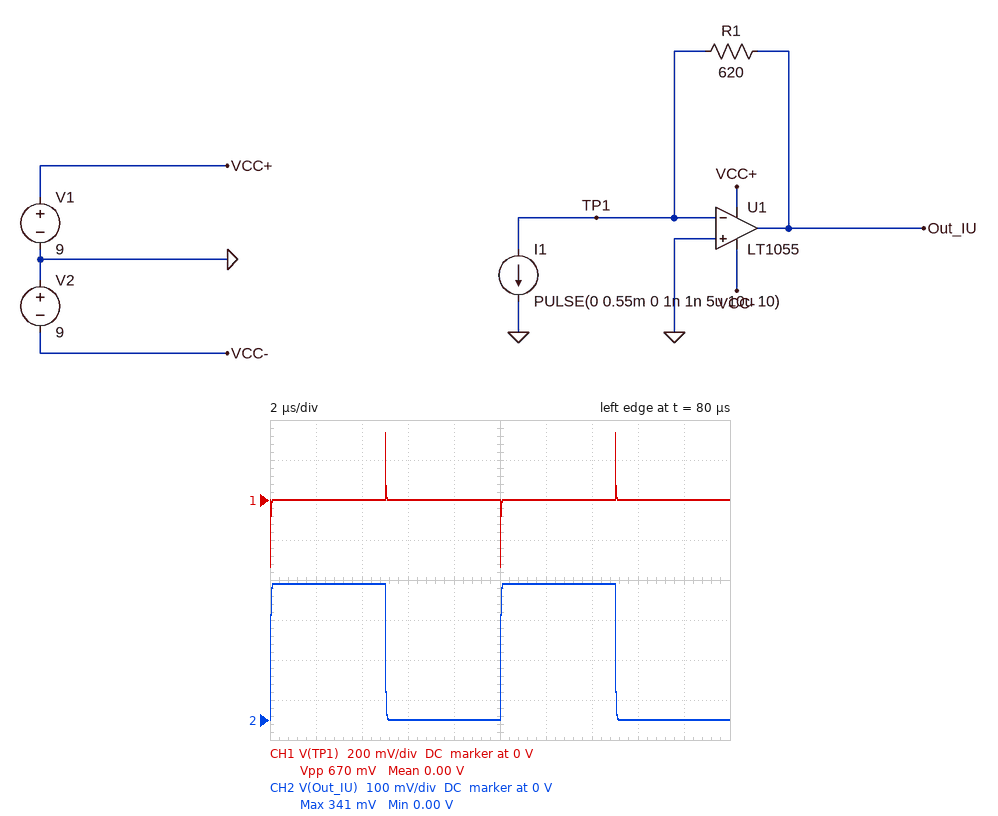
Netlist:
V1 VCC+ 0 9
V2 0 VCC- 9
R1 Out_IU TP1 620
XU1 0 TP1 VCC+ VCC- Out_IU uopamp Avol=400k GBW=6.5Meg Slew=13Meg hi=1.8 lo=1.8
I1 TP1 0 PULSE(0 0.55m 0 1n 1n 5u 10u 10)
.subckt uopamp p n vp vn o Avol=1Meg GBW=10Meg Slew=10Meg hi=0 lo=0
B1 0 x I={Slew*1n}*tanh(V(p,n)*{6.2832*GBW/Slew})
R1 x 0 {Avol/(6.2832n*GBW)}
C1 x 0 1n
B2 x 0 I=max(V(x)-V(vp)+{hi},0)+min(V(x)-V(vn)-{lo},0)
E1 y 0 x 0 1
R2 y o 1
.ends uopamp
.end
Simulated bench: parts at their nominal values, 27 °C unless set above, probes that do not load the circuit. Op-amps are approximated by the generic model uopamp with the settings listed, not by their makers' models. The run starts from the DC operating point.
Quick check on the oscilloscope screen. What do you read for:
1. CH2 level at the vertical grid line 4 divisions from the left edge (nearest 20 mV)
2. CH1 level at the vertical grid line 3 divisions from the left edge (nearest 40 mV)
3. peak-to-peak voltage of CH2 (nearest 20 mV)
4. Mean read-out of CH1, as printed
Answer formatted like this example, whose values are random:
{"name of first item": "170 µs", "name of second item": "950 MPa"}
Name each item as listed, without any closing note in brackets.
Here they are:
{"CH2 level at the vertical grid line 4 divisions from the left edge": "0 V", "CH1 level at the vertical grid line 3 divisions from the left edge": "0 V", "peak-to-peak voltage of CH2": "340 mV", "Mean read-out of CH1, as printed": "0.00 V"}
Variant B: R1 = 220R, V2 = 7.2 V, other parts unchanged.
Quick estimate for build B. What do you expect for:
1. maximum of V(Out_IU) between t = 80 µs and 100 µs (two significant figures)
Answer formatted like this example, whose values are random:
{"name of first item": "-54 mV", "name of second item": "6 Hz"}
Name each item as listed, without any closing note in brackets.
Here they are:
{"maximum of V(Out_IU) between t = 80 µs and 100 µs": "120 mV"}
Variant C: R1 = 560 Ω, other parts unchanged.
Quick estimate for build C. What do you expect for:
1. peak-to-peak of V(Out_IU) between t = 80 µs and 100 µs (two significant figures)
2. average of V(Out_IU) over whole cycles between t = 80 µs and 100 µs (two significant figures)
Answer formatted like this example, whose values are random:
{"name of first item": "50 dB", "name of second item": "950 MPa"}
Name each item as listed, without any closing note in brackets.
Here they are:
{"peak-to-peak of V(Out_IU) between t = 80 µs and 100 µs": "310 mV", "average of V(Out_IU) over whole cycles between t = 80 µs and 100 µs": "150 mV"}
